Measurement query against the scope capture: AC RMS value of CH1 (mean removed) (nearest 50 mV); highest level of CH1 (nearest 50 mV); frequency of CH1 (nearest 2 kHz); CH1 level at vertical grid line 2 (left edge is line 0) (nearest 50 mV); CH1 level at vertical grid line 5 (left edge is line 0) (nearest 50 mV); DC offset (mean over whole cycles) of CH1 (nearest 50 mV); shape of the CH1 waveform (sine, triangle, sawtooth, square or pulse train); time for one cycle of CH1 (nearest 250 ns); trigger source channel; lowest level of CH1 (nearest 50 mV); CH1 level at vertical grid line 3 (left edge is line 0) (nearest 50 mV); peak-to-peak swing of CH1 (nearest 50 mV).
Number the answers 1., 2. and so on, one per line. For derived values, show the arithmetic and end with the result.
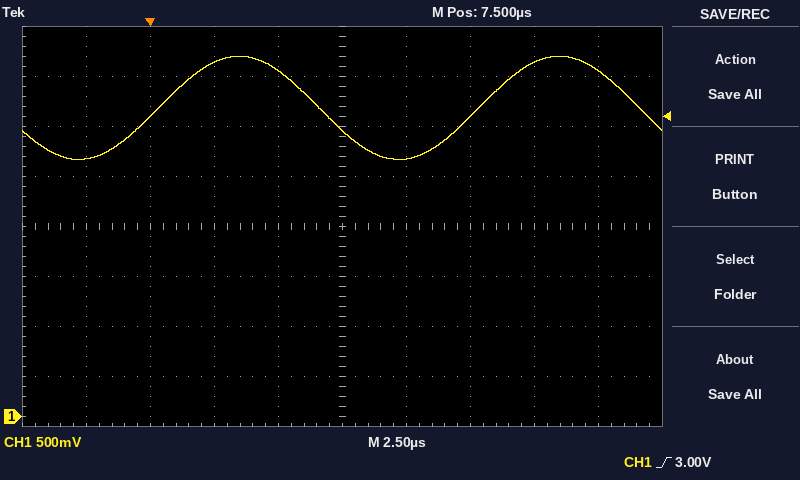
1. 1.05 V / (2√2) ≈ 371 mV, so 350 mV to the nearest 50 mV
2. 3.60 V
3. 1 / 12.50 µs ≈ 80 kHz
4. 3.00 V
5. 2.85 V
6. (3.60 V + (2.55 V)) / 2 ≈ 3.08 V, so 3.10 V to the nearest 50 mV
7. sine
8. 12.50 µs
9. CH1
10. 2.55 V
11. 3.55 V
12. 3.60 V − (2.55 V) = 1.05 V
